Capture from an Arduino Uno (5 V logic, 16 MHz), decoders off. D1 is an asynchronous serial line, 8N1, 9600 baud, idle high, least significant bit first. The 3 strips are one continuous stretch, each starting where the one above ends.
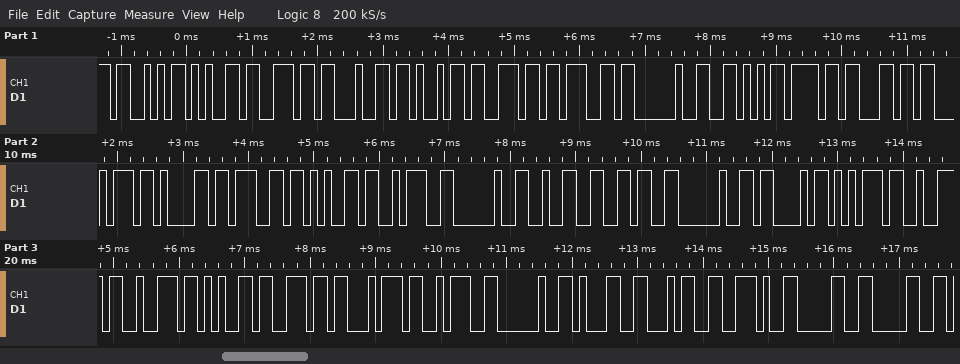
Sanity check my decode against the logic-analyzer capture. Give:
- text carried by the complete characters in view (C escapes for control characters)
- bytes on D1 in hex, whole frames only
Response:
"Sending Voltage: 26 Current: 14.00"
53 65 6E 64 69 6E 67 20 56 6F 6C 74 61 67 65 3A 20 32 36 20 43 75 72 72 65 6E 74 3A 20 31 34 2E 30 30
